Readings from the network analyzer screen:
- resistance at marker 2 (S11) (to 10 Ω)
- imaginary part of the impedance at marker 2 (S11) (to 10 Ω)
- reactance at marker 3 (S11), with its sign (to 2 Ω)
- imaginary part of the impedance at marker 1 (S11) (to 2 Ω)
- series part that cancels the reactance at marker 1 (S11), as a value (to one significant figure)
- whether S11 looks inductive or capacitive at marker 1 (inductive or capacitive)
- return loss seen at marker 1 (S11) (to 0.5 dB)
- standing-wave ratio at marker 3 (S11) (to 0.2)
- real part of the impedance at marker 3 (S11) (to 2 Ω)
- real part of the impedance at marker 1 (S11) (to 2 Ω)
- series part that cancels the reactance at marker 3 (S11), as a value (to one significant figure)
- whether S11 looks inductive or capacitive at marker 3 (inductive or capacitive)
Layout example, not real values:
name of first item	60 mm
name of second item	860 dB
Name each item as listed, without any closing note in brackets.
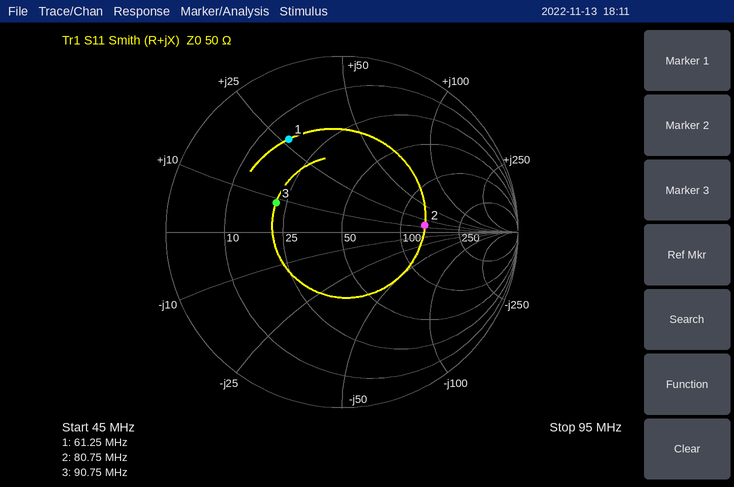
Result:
resistance at marker 2 (S11)	140 Ω
imaginary part of the impedance at marker 2 (S11)	+10 Ω
reactance at marker 3 (S11), with its sign	+8 Ω
imaginary part of the impedance at marker 1 (S11)	+26 Ω
series part that cancels the reactance at marker 1 (S11), as a value	100 pF
whether S11 looks inductive or capacitive at marker 1	inductive
return loss seen at marker 1 (S11)	4.5 dB
standing-wave ratio at marker 3 (S11)	2.4
real part of the impedance at marker 3 (S11)	22 Ω
real part of the impedance at marker 1 (S11)	16 Ω
series part that cancels the reactance at marker 3 (S11), as a value	200 pF
whether S11 looks inductive or capacitive at marker 3	inductive
